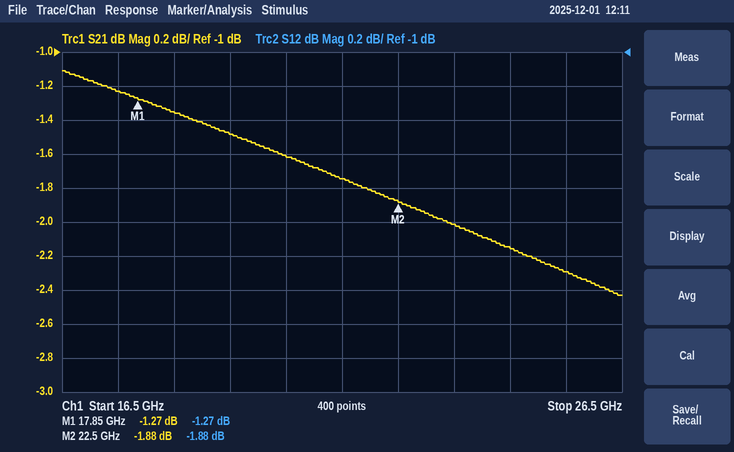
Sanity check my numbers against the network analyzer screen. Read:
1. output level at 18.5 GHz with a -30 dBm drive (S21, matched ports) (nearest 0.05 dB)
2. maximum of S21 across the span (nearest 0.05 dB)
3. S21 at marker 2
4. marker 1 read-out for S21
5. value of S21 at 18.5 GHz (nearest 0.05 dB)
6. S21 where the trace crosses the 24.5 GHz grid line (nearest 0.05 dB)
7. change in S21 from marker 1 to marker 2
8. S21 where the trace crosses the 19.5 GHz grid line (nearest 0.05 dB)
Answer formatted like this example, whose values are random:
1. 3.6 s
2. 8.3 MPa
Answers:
1. -31.35 dBm
2. -1.10 dB
3. -1.88 dB
4. -1.27 dB
5. -1.35 dB
6. -2.15 dB
7. -0.61 dB
8. -1.50 dB
